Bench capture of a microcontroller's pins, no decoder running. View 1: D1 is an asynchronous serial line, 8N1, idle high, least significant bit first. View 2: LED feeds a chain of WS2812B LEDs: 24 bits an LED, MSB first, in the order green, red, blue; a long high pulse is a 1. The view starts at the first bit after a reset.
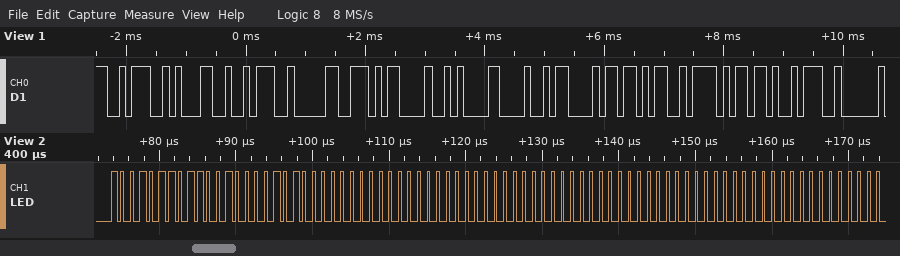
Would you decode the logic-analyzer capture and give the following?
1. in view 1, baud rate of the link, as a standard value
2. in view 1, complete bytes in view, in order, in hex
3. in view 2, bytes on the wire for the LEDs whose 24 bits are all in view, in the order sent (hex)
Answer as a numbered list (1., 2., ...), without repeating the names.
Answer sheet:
1. 9600 baud
2. 3A 31 3A 30 0D 0A 48 68 4D 6D 3A
3. 96 C8 50 00 00 00 00 00 00
